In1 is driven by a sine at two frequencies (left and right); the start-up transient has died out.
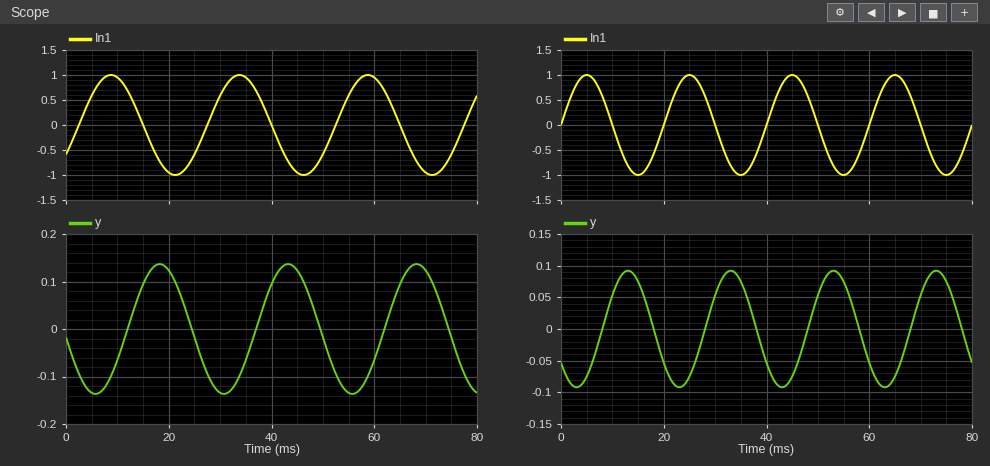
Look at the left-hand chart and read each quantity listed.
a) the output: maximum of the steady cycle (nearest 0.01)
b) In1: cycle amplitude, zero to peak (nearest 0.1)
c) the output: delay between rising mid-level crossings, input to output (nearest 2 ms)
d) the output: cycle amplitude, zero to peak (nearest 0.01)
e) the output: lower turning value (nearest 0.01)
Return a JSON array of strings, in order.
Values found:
["0.14", "1.0", "10 ms", "0.14", "-0.14"]
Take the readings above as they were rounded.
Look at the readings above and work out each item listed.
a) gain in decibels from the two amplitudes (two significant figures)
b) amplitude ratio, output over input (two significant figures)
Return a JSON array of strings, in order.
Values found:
["-17 dB", "0.14"]
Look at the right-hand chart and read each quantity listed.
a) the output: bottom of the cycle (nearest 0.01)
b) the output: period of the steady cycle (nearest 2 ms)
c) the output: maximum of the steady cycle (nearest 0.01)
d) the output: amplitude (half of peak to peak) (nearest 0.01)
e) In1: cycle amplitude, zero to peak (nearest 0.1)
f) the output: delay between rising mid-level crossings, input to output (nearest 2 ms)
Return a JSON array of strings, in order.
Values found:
["-0.09", "20 ms", "0.09", "0.09", "1.0", "8 ms"]
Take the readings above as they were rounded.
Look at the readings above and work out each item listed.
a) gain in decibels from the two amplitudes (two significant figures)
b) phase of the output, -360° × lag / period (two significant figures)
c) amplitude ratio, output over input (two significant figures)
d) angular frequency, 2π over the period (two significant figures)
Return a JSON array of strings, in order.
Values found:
["-21 dB", "-140°", "0.090", "0.31 rad/ms"]
